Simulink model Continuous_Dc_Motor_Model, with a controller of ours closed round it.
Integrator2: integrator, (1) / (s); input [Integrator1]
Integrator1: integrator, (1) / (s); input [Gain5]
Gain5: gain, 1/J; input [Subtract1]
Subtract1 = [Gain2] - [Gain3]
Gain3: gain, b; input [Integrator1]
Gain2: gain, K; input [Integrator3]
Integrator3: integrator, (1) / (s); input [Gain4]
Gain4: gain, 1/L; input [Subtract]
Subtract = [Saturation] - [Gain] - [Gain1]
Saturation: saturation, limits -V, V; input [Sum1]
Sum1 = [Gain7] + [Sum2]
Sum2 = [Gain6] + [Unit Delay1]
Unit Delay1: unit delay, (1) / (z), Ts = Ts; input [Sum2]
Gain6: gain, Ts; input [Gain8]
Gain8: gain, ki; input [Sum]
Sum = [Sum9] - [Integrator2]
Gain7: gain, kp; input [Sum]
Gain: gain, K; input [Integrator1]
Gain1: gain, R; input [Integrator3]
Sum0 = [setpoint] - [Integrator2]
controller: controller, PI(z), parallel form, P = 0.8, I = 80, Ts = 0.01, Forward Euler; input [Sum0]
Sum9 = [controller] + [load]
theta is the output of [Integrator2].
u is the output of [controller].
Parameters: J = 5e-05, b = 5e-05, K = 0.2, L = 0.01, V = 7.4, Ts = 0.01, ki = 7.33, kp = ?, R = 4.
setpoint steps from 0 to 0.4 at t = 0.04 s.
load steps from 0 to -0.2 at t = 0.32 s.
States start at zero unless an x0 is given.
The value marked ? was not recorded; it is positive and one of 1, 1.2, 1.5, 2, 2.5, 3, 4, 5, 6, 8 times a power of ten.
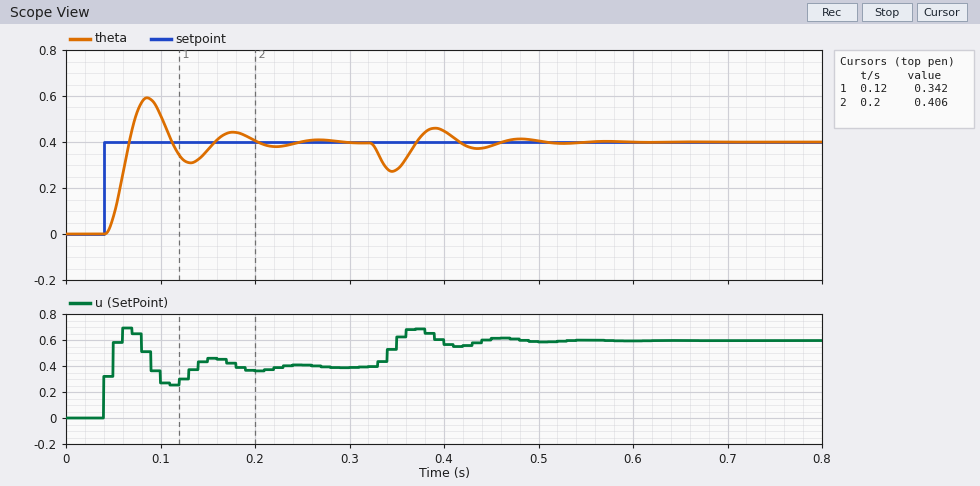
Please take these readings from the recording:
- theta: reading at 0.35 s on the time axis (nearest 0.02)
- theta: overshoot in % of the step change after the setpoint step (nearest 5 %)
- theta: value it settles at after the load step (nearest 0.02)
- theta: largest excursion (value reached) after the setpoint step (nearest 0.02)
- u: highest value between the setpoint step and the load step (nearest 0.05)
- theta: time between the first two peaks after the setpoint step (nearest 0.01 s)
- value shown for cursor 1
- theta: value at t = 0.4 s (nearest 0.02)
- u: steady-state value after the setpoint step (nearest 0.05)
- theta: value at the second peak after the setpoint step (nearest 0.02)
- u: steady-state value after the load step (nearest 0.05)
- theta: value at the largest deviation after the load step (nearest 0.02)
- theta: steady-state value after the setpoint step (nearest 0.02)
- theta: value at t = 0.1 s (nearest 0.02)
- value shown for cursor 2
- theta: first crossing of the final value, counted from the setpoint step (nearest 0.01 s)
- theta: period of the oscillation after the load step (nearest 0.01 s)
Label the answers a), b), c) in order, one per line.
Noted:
a) 0.28
b) 50 %
c) 0.40
d) 0.60
e) 0.70
f) 0.09 s
g) 0.342
h) 0.44
i) 0.40
j) 0.44
k) 0.60
l) 0.28
m) 0.40
n) 0.52
o) 0.406
p) 0.03 s
q) 0.09 s
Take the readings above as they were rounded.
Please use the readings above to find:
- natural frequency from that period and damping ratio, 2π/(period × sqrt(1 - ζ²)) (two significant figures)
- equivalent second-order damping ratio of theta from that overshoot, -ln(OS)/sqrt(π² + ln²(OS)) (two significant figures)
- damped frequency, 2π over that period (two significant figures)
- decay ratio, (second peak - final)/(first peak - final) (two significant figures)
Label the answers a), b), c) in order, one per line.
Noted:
a) 72 rad/s
b) 0.22
c) 70 rad/s
d) 0.20
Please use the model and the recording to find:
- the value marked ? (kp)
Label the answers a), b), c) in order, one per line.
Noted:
a) 10
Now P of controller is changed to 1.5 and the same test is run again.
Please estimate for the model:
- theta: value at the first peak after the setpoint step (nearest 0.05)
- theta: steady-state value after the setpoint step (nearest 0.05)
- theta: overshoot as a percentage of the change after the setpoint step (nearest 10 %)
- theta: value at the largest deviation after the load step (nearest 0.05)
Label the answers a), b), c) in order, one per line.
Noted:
a) 0.55
b) 0.40
c) 30 %
d) 0.30
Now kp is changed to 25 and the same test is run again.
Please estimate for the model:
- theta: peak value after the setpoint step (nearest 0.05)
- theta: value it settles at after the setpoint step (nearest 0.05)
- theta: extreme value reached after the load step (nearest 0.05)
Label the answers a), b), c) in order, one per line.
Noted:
a) 0.55
b) 0.40
c) 0.20
